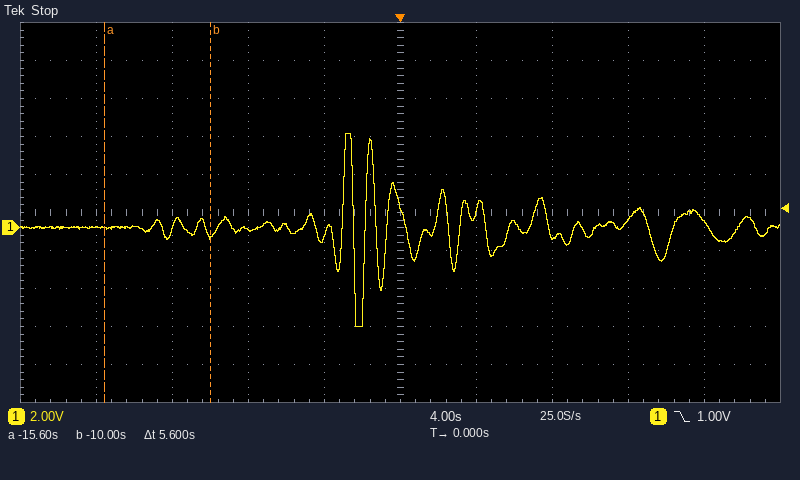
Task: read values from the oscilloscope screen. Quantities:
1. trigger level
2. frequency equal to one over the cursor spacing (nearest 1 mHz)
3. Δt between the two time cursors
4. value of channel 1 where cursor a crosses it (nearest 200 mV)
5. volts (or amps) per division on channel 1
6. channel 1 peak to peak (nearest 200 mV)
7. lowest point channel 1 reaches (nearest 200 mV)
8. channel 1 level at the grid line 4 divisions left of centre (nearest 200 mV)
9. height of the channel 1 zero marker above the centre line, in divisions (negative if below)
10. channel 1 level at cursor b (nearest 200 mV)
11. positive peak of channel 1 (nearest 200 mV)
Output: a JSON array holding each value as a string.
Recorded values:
["1.00 V", "179 mHz", "5.6 s", "0.0 V", "2 V", "10.2 V", "-5.2 V", "0.0 V", "-0.4 div", "-400 mV", "5.0 V"]
